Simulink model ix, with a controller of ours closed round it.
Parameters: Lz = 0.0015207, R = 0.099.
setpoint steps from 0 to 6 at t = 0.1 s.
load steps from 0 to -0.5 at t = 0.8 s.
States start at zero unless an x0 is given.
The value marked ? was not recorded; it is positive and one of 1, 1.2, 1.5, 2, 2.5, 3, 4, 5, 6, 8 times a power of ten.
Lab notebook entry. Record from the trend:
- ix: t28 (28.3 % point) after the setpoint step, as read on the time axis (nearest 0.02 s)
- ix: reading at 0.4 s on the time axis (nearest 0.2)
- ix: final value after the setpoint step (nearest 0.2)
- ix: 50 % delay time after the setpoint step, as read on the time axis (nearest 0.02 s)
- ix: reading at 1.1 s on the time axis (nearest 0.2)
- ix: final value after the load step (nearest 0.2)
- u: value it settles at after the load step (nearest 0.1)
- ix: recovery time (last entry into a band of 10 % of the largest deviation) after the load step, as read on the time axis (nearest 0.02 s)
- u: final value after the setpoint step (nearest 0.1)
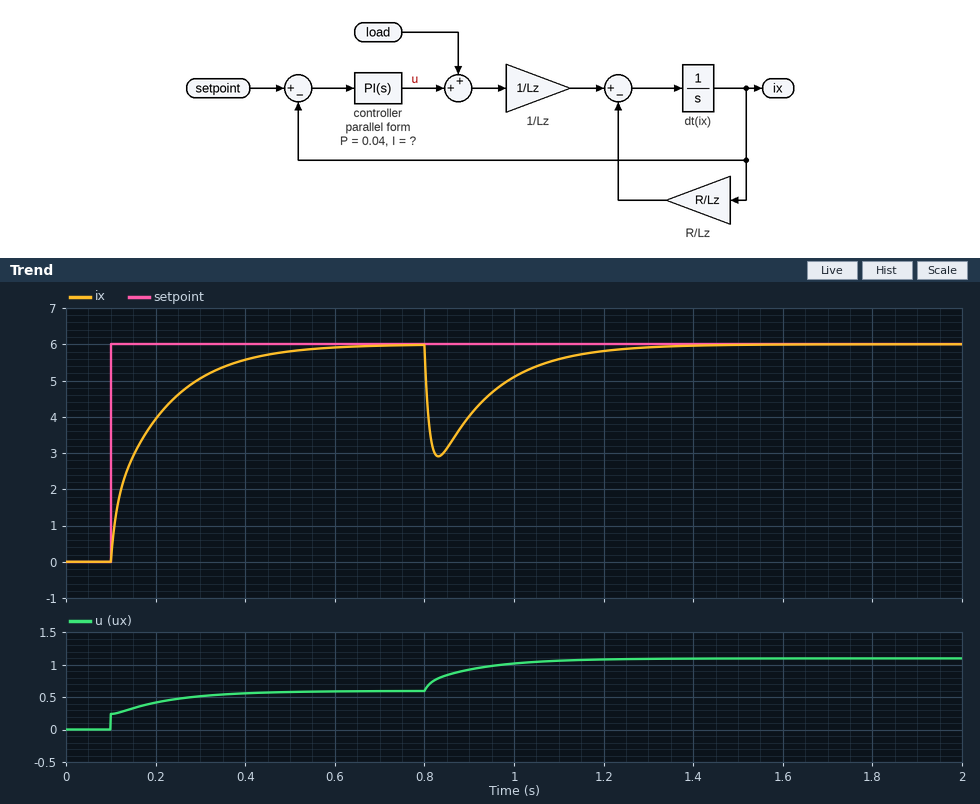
0.12 s
5.6
6.0
0.16 s
5.6
6.0
1.1
1.14 s
0.6
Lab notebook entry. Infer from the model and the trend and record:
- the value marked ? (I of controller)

1
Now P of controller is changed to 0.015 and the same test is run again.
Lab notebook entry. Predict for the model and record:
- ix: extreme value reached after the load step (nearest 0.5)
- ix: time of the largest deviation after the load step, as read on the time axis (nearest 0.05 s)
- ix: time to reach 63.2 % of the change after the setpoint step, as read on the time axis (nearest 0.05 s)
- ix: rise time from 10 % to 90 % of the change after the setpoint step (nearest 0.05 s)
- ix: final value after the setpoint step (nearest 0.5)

2.5
0.85 s
0.20 s
0.20 s
6.0
